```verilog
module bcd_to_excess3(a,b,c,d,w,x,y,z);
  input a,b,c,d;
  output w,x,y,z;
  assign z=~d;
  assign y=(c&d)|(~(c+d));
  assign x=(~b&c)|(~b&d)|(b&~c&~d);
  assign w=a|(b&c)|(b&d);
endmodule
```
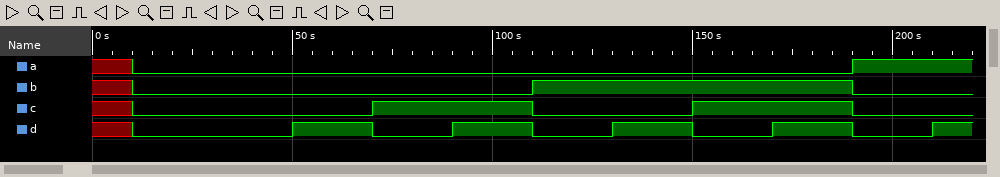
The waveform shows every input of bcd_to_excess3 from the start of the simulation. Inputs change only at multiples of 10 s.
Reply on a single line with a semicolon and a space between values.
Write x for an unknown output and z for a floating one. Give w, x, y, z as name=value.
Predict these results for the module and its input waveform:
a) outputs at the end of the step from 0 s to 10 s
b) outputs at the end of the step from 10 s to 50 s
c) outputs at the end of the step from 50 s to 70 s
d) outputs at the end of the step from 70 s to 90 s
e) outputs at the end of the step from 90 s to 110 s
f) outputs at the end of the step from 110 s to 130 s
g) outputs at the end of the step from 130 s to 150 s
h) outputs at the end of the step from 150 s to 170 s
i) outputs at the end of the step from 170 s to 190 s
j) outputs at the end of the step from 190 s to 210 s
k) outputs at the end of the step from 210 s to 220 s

w=x, x=x, y=x, z=x; w=0, x=0, y=1, z=1; w=0, x=1, y=0, z=0; w=0, x=1, y=0, z=1; w=0, x=1, y=1, z=0; w=0, x=1, y=1, z=1; w=1, x=0, y=0, z=0; w=1, x=0, y=0, z=1; w=1, x=0, y=1, z=0; w=1, x=0, y=1, z=1; w=1, x=1, y=0, z=0
